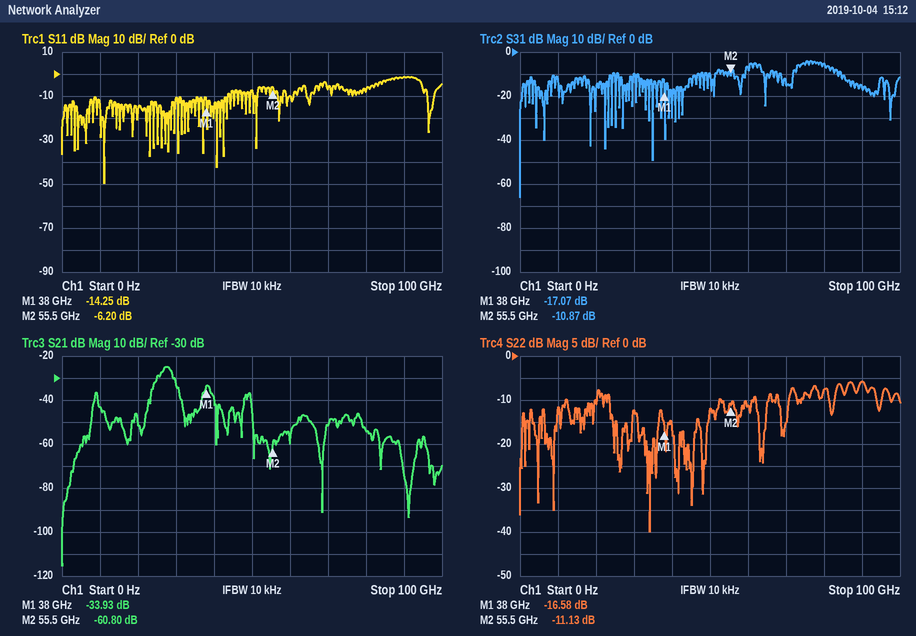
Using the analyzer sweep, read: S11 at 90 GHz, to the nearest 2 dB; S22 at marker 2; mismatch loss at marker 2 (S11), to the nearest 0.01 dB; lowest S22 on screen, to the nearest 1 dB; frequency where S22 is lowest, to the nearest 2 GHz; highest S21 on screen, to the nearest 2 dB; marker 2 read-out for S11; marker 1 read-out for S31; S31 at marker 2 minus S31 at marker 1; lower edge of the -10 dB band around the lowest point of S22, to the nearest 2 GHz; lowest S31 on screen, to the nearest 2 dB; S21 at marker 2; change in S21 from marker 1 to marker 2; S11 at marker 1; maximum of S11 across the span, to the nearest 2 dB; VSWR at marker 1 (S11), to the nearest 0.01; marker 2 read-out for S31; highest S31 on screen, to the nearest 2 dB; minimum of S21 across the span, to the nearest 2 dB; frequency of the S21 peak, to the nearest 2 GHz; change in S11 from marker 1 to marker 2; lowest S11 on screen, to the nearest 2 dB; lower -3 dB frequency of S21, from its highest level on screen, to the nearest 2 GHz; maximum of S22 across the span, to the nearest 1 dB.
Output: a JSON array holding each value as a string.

["-2 dB", "-11.13 dB", "1.19 dB", "-40 dB", "34 GHz", "-24 dB", "-6.20 dB", "-17.07 dB", "6.20 dB", "24 GHz", "-66 dB", "-60.80 dB", "-26.87 dB", "-14.25 dB", "-2 dB", "1.48", "-10.87 dB", "-4 dB", "-116 dB", "28 GHz", "8.05 dB", "-50 dB", "26 GHz", "-6 dB"]
